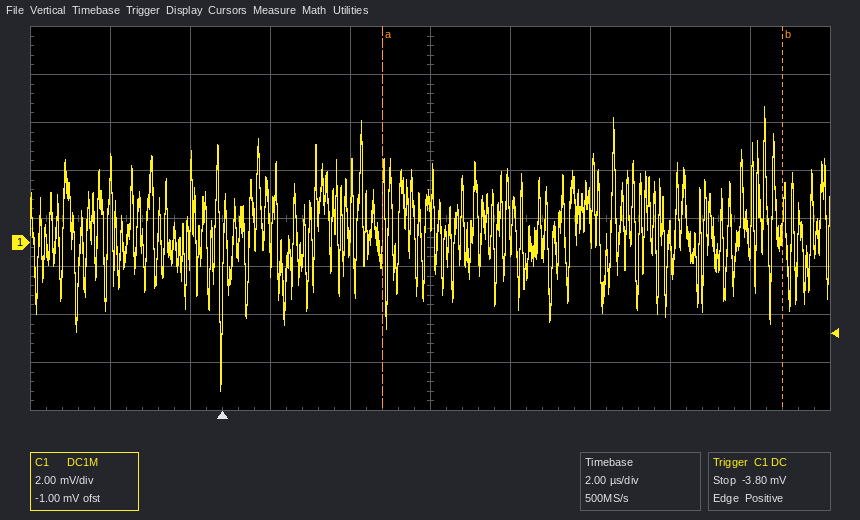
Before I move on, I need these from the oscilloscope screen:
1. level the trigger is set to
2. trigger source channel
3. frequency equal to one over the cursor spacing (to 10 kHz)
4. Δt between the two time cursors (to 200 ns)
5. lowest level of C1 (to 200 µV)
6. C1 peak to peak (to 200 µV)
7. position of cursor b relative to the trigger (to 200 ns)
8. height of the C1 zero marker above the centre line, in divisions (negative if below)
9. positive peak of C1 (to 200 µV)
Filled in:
-3.80 mV
C1
100 kHz
10.0 µs
-6.2 mV
11.8 mV
+14.0 µs
-0.5 div
5.6 mV
